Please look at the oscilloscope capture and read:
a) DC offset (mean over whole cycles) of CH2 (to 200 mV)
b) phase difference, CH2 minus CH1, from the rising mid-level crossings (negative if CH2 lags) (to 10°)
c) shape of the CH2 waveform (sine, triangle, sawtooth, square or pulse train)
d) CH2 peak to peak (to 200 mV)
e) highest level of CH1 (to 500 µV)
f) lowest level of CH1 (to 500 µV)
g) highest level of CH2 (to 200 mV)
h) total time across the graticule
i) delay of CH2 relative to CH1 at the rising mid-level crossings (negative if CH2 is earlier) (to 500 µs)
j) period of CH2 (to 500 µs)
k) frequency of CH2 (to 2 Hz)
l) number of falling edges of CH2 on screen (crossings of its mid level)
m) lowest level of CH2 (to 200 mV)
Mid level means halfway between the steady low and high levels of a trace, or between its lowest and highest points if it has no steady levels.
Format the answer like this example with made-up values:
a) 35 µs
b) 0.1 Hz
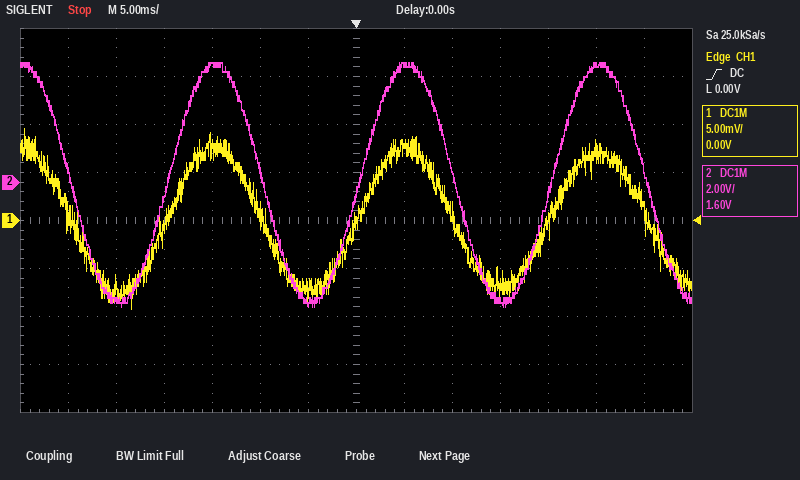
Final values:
a) 0.0 V
b) 0°
c) sine
d) 10.2 V
e) 9.5 mV
f) -9.0 mV
g) 5.0 V
h) 70 ms
i) 0.0 ms
j) 20.0 ms
k) 50 Hz
l) 4
m) -5.2 V
